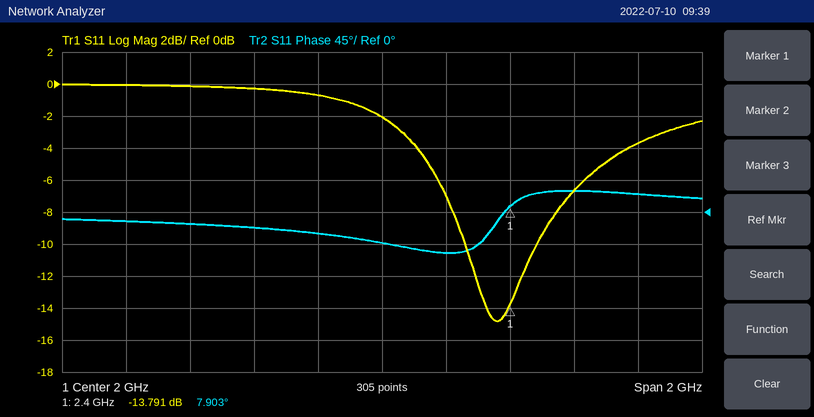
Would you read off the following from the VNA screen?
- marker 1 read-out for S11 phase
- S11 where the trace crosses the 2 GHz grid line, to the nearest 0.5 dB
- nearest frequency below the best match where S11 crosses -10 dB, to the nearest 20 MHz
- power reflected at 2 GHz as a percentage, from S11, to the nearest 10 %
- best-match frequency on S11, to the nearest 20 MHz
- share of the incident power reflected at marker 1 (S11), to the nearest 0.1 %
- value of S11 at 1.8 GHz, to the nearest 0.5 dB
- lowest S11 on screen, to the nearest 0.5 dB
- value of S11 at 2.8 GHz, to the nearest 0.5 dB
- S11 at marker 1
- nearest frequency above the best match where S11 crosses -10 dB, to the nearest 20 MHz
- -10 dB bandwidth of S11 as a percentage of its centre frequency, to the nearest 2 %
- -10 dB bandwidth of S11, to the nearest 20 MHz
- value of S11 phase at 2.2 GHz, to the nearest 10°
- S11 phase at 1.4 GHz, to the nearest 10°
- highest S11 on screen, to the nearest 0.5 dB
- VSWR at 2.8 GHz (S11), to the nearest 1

7.903°
-2.0 dB
2.26 GHz
60 %
2.36 GHz
4.2 %
-0.5 dB
-15.0 dB
-3.5 dB
-13.791 dB
2.48 GHz
10 %
220 MHz
-60°
-20°
0.0 dB
5
